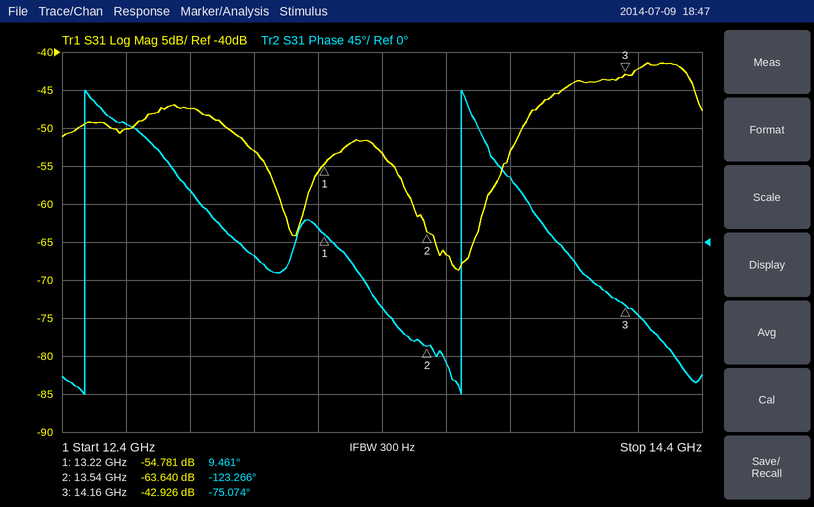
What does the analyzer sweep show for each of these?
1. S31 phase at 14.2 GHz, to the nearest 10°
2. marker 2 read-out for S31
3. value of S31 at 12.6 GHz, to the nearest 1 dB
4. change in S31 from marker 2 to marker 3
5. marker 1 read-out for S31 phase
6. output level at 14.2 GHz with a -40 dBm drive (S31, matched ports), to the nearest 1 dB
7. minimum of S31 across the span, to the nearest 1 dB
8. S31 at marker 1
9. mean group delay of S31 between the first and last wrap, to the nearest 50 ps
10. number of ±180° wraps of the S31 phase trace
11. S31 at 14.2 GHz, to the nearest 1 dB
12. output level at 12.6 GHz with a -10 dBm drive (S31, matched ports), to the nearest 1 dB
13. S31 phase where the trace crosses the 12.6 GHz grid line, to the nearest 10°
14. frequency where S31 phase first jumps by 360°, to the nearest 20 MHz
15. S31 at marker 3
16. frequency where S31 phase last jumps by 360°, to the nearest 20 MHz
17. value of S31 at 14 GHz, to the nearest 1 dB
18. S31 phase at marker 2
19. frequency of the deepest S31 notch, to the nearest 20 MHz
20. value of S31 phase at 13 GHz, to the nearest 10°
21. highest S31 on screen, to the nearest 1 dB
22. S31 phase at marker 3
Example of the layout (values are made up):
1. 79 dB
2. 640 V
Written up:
1. -90°
2. -63.640 dB
3. -50 dB
4. 20.714 dB
5. 9.461°
6. -82 dBm
7. -69 dB
8. -54.781 dB
9. 850 ps
10. 2
11. -42 dB
12. -60 dBm
13. 140°
14. 12.48 GHz
15. -42.926 dB
16. 13.64 GHz
17. -44 dB
18. -123.266°
19. 13.64 GHz
20. -20°
21. -41 dB
22. -75.074°
